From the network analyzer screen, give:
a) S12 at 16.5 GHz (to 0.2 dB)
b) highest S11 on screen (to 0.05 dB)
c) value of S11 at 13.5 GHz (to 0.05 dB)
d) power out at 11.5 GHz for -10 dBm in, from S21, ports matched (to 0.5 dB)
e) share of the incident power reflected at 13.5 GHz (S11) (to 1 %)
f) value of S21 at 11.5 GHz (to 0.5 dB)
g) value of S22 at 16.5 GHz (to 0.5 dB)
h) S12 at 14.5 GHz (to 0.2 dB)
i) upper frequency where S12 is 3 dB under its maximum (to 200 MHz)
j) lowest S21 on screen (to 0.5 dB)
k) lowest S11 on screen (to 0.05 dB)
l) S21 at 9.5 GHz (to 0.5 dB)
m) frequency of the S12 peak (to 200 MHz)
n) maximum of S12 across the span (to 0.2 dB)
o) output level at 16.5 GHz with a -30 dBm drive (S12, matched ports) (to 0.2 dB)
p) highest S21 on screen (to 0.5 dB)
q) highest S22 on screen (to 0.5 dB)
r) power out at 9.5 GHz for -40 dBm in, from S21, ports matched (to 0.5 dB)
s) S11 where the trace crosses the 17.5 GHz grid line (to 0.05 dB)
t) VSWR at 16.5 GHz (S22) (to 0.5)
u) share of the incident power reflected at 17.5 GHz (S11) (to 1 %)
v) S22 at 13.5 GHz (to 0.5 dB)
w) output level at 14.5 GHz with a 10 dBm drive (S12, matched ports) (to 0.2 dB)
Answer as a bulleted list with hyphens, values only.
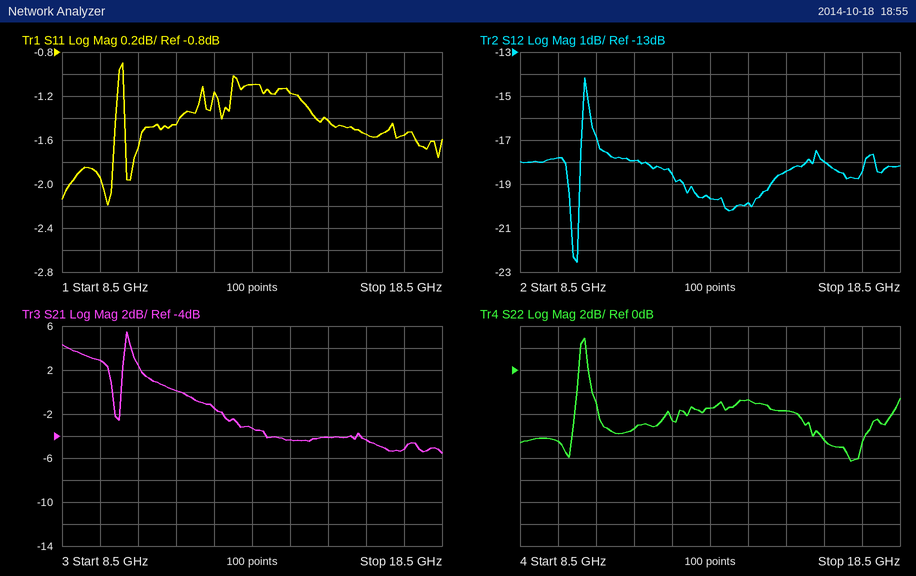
- -18.0 dB
- -0.90 dB
- -1.10 dB
- -10.0 dBm
- 78 %
- 0.0 dB
- -6.5 dB
- -19.8 dB
- 10.6 GHz
- -5.5 dB
- -2.20 dB
- 3.0 dB
- 10.2 GHz
- -14.2 dB
- -48.0 dBm
- 5.5 dB
- 3.0 dB
- -37.0 dBm
- -1.55 dB
- 3.0
- 70 %
- -3.5 dB
- -9.8 dBm
